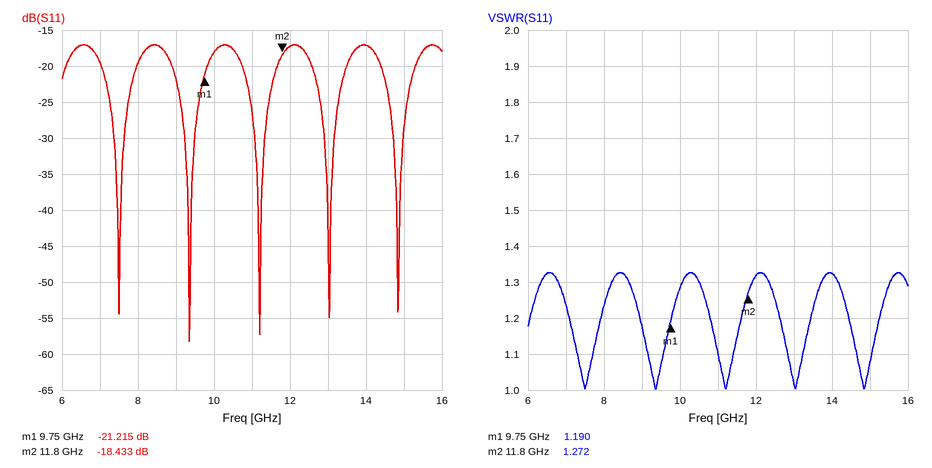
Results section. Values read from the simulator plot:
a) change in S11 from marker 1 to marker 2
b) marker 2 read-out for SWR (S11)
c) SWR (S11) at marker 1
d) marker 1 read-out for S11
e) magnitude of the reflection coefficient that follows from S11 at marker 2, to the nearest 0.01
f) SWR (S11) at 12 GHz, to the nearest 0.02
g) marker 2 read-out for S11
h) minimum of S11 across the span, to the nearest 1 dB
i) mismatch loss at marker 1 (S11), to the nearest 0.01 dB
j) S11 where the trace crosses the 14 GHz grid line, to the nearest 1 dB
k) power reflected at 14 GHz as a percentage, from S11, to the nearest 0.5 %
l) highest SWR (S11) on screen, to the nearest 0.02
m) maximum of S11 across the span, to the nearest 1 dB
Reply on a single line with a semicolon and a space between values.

2.782 dB; 1.272; 1.190; -21.215 dB; 0.12; 1.32; -18.433 dB; -58 dB; 0.03 dB; -17 dB; 2.0 %; 1.32; -17 dB
